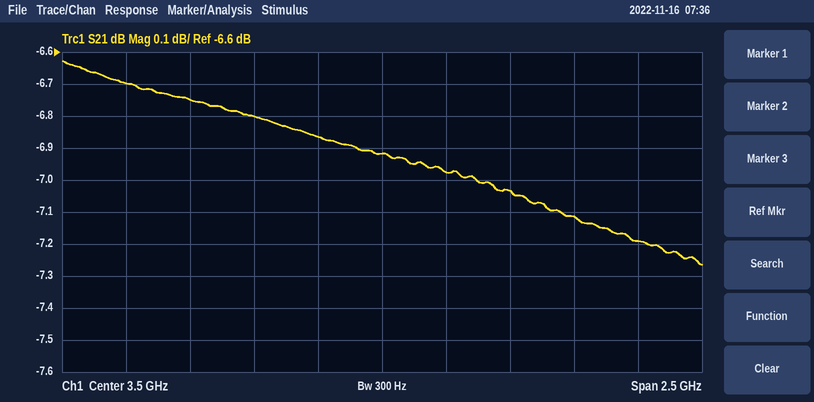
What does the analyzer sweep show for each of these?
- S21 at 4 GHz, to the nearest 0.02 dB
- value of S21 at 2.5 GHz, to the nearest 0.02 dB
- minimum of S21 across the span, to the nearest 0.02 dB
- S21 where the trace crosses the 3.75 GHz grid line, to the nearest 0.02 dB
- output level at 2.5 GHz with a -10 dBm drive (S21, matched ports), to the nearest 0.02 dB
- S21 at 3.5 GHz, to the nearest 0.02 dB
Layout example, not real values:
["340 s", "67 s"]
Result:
["-7.04 dB", "-6.70 dB", "-7.26 dB", "-6.98 dB", "-16.70 dBm", "-6.92 dB"]
